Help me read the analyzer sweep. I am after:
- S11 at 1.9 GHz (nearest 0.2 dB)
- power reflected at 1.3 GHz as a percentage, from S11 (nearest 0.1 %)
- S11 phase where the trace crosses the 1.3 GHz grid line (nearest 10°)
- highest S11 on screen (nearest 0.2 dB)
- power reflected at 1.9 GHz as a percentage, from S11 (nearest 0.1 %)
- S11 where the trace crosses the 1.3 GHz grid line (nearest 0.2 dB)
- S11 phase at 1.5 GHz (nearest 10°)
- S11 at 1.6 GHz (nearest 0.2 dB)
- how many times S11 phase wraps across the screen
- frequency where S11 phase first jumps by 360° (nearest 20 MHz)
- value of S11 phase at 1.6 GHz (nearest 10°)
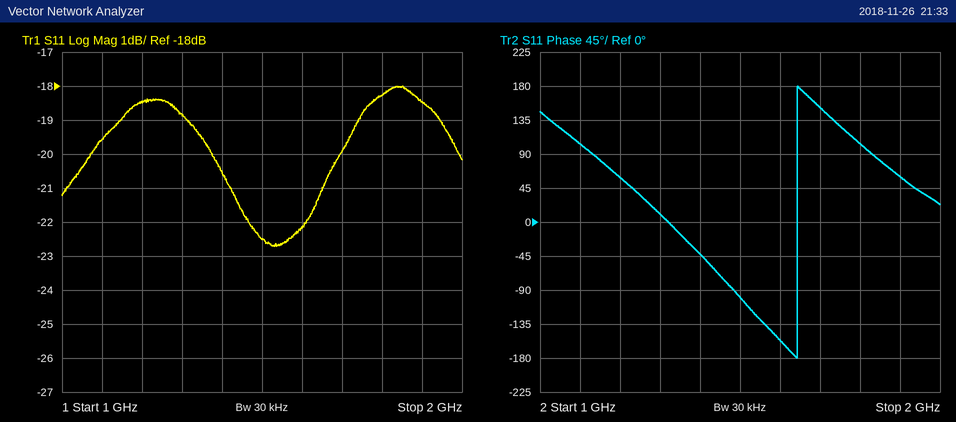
-18.4 dB
1.3 %
10°
-18.0 dB
1.4 %
-18.8 dB
-100°
-22.2 dB
1
1.64 GHz
-160°
